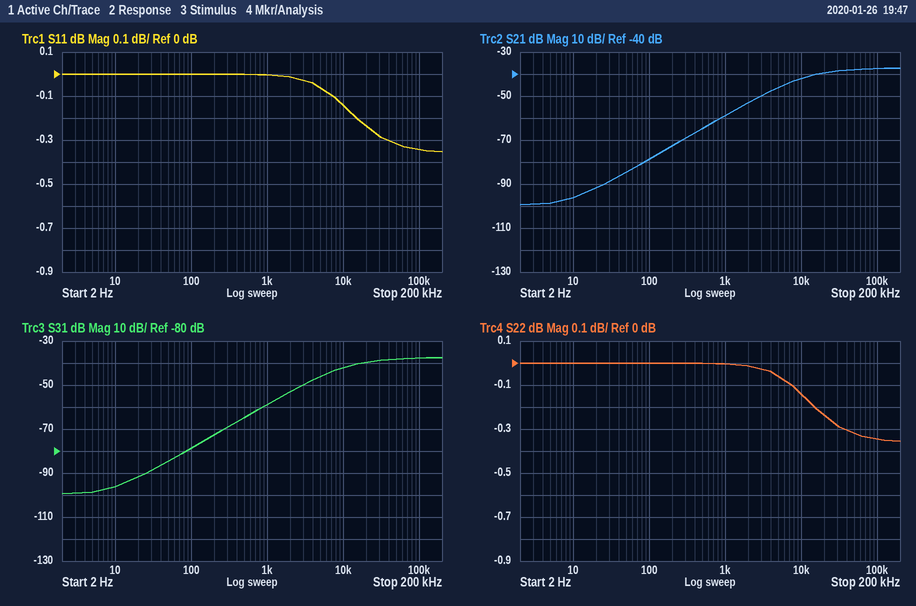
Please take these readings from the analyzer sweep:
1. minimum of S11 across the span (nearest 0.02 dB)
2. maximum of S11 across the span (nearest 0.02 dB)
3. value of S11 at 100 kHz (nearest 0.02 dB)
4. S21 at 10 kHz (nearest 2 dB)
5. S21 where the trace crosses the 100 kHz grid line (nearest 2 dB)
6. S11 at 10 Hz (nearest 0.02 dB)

-0.36 dB
0.00 dB
-0.34 dB
-42 dB
-38 dB
0.00 dB
